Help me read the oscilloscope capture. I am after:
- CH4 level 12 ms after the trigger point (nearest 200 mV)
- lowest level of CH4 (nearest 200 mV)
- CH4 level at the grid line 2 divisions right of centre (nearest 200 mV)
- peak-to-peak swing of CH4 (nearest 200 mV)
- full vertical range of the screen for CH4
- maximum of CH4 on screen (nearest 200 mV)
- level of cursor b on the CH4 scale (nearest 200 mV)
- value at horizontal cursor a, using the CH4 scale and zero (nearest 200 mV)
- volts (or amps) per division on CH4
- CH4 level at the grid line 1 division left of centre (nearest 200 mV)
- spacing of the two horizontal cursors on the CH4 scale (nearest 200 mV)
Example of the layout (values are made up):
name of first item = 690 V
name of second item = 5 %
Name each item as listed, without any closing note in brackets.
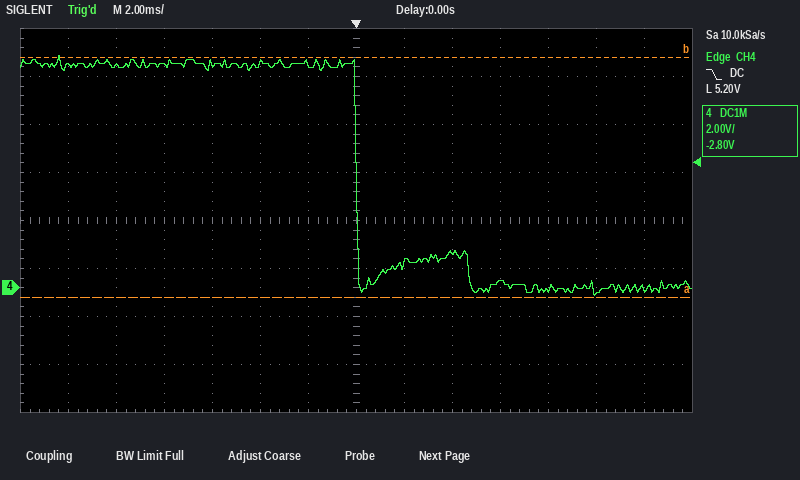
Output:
CH4 level 12 ms after the trigger point = 0.0 V
lowest level of CH4 = -400 mV
CH4 level at the grid line 2 divisions right of centre = 1.4 V
peak-to-peak swing of CH4 = 10.0 V
full vertical range of the screen for CH4 = 16 V
maximum of CH4 on screen = 9.6 V
level of cursor b on the CH4 scale = 9.6 V
value at horizontal cursor a, using the CH4 scale and zero = -400 mV
volts (or amps) per division on CH4 = 2 V
CH4 level at the grid line 1 division left of centre = 9.4 V
spacing of the two horizontal cursors on the CH4 scale = 10.0 V
